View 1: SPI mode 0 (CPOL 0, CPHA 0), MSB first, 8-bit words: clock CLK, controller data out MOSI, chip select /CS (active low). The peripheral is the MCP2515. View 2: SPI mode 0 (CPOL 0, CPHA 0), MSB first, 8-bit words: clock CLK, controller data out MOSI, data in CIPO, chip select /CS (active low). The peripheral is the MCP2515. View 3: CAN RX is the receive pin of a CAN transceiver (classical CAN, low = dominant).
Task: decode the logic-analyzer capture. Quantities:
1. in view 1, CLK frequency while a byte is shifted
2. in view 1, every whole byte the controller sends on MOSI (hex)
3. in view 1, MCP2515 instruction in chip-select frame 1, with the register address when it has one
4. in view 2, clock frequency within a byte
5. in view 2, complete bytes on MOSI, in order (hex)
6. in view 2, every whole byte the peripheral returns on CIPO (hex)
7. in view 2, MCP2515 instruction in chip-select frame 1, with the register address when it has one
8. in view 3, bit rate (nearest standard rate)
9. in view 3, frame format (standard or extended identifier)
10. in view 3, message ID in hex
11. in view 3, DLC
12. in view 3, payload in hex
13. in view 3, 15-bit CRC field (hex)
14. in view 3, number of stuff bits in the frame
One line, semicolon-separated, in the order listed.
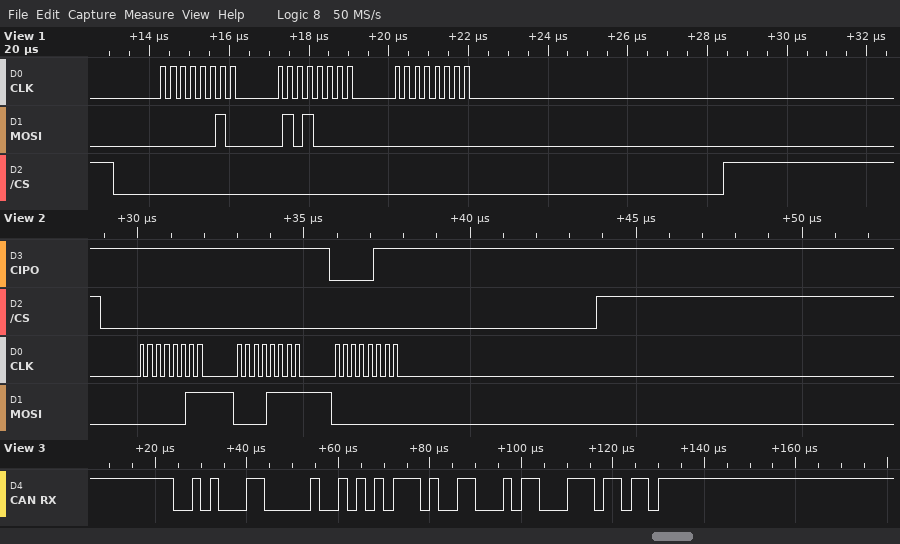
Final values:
4 MHz; 02 50 00; WRITE 0x50; 4 MHz; 03 0F 00; FF FF 07; READ 0x0F; 500 kbit/s; standard; 0x28C; 2; AE 98; 0x58ED; 1
